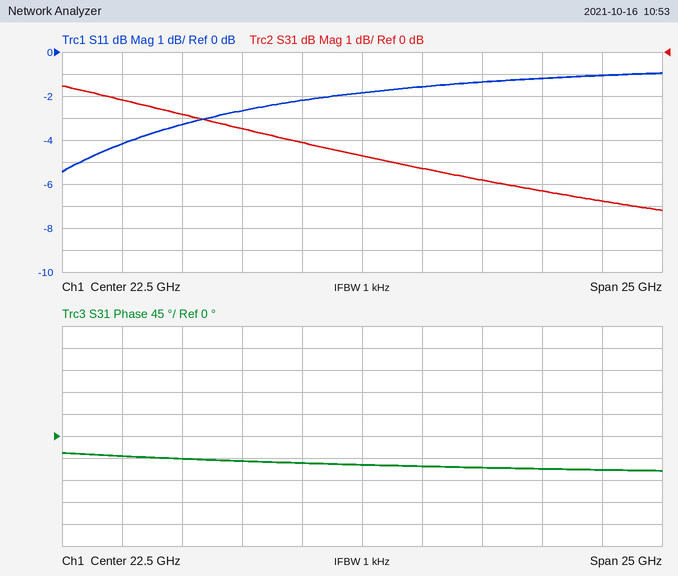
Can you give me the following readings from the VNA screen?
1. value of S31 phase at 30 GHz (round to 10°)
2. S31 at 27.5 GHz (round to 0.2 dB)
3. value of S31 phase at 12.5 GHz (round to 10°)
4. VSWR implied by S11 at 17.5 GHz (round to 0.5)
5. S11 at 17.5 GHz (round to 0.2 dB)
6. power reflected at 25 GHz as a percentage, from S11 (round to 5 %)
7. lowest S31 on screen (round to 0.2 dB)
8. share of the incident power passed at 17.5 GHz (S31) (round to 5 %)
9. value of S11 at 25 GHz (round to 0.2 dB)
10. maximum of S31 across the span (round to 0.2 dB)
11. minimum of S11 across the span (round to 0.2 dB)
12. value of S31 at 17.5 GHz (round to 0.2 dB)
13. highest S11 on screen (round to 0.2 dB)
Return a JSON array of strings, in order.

["-70°", "-5.8 dB", "-40°", "6.5", "-2.6 dB", "70 %", "-7.2 dB", "45 %", "-1.6 dB", "-1.6 dB", "-5.4 dB", "-3.4 dB", "-1.0 dB"]
